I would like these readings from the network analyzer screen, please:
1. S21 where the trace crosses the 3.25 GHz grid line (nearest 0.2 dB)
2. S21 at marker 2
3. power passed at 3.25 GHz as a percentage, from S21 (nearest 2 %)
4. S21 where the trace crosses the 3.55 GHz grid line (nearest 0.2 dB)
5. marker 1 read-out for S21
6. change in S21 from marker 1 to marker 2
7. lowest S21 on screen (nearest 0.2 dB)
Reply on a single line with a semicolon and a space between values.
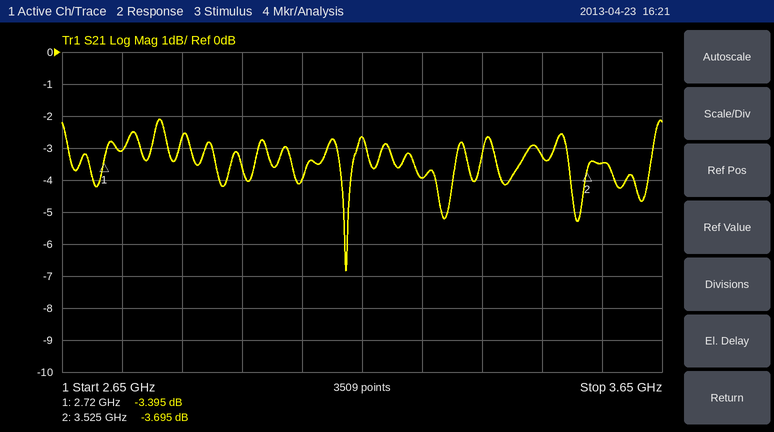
-4.0 dB; -3.695 dB; 40 %; -3.4 dB; -3.395 dB; -0.300 dB; -6.8 dB
